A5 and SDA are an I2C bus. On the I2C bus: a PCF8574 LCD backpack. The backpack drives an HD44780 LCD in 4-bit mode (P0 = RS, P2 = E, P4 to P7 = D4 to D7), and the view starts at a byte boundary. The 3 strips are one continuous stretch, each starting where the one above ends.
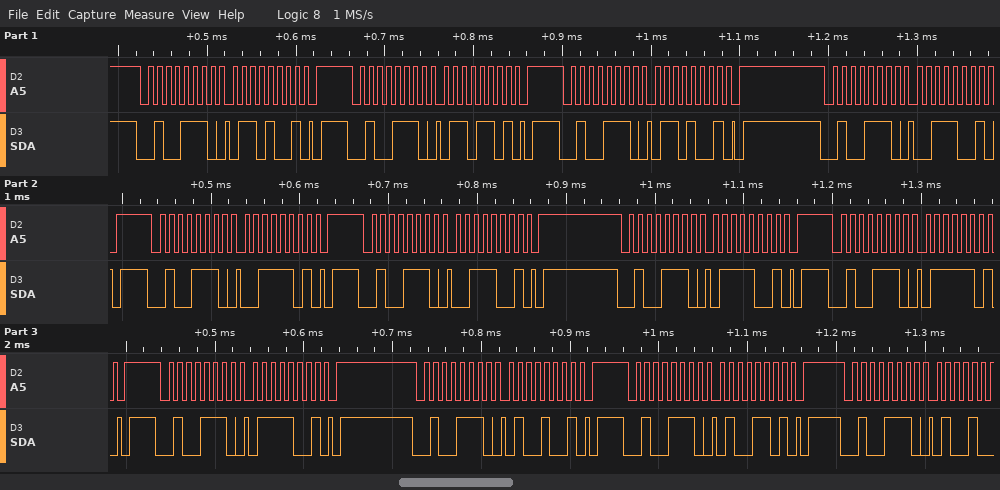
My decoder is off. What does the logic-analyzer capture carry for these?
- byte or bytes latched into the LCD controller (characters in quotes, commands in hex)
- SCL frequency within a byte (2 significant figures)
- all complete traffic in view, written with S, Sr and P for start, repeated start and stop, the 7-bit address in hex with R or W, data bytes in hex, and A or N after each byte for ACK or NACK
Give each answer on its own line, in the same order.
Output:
'c'
100 kHz
S 27W A 69 A P S 27W A 6D A P S 27W A 69 A P S 27W A 39 A P S 27W A 3D A P S 27W A 39 A P S 27W A 79 A P S 27W A 7D A P S 27W A 79 A P S 27W A 49 A P S 27W A 4D A P S 27W A
